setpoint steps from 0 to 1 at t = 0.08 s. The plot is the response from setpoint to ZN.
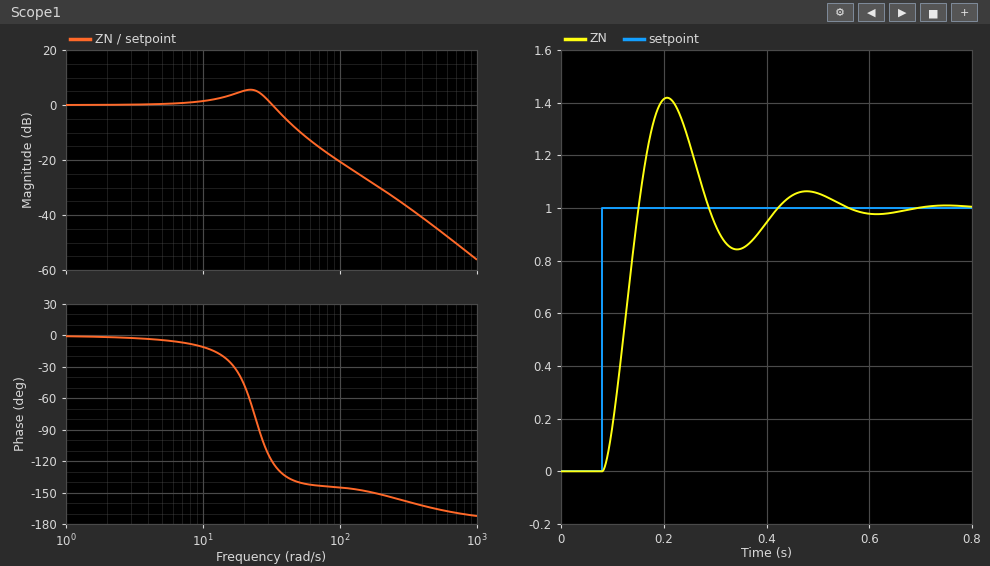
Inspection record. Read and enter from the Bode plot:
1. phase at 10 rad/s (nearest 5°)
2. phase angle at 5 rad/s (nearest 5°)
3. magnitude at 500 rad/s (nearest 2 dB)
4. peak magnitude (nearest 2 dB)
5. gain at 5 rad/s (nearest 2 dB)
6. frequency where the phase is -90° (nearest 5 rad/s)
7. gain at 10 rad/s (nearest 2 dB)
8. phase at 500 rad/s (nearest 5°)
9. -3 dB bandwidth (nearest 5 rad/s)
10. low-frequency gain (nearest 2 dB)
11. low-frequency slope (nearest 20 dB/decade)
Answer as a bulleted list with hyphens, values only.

- -10°
- -5°
- -44 dB
- 6 dB
- 0 dB
- 25 rad/s
- 2 dB
- -165°
- 35 rad/s
- 0 dB
- 0 dB/decade
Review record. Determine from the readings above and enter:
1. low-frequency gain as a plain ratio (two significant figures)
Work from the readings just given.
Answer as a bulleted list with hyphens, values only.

- 1.0
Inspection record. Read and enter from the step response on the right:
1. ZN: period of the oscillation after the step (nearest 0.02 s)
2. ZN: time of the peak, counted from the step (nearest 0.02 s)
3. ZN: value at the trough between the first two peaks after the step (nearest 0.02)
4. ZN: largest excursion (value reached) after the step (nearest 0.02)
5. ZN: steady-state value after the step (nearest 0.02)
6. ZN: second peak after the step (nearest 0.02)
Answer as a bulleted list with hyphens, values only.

- 0.28 s
- 0.12 s
- 0.84
- 1.42
- 1.00
- 1.06
